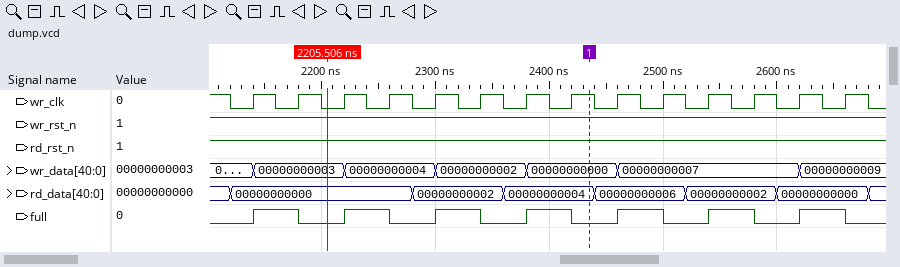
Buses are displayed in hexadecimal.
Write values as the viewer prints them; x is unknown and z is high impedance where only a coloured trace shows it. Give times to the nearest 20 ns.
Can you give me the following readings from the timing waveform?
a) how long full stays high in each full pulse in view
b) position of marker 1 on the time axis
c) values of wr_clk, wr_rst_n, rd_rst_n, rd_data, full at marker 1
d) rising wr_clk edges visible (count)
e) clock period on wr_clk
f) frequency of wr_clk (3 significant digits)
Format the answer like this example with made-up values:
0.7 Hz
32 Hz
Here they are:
40 ns, 40 ns, 40 ns, 40 ns, 40 ns, 40 ns, 40 ns
2440 ns
wr_clk=1, wr_rst_n=1, rd_rst_n=1, rd_data=00000000004, full=0
14
40 ns
25.0 MHz
